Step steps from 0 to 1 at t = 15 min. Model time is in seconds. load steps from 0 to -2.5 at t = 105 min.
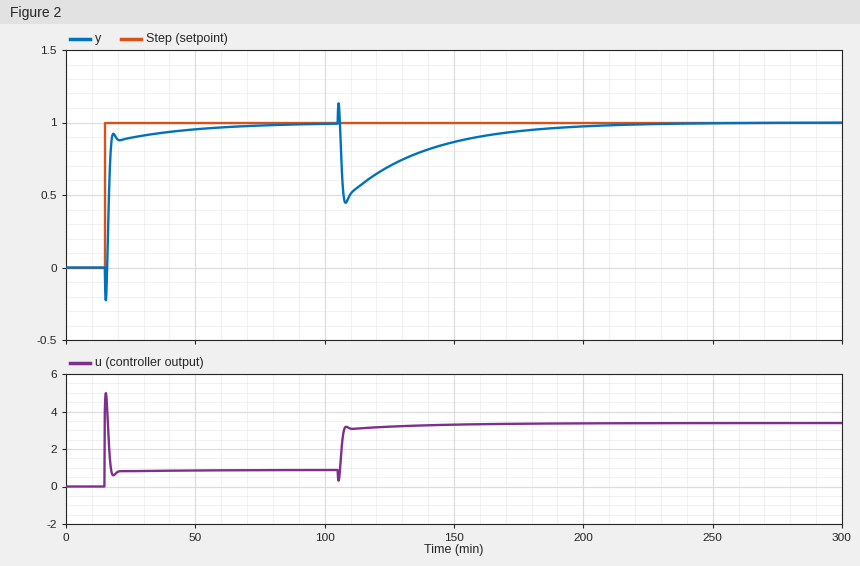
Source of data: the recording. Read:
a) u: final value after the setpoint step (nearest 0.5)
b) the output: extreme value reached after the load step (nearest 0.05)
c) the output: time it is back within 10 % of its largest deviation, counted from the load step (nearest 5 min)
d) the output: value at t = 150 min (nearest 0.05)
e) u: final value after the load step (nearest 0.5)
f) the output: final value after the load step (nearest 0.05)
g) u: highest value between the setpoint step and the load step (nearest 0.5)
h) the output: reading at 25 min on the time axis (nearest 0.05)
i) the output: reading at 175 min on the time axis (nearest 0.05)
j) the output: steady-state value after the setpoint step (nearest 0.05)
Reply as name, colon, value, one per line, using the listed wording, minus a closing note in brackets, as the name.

u: final value after the setpoint step: 1.0
the output: extreme value reached after the load step: 0.45
the output: time it is back within 10 % of its largest deviation, counted from the load step: 75 min
the output: value at t = 150 min: 0.85
u: final value after the load step: 3.5
the output: final value after the load step: 1.00
u: highest value between the setpoint step and the load step: 5.0
the output: reading at 25 min on the time axis: 0.90
the output: reading at 175 min on the time axis: 0.95
the output: steady-state value after the setpoint step: 1.00
